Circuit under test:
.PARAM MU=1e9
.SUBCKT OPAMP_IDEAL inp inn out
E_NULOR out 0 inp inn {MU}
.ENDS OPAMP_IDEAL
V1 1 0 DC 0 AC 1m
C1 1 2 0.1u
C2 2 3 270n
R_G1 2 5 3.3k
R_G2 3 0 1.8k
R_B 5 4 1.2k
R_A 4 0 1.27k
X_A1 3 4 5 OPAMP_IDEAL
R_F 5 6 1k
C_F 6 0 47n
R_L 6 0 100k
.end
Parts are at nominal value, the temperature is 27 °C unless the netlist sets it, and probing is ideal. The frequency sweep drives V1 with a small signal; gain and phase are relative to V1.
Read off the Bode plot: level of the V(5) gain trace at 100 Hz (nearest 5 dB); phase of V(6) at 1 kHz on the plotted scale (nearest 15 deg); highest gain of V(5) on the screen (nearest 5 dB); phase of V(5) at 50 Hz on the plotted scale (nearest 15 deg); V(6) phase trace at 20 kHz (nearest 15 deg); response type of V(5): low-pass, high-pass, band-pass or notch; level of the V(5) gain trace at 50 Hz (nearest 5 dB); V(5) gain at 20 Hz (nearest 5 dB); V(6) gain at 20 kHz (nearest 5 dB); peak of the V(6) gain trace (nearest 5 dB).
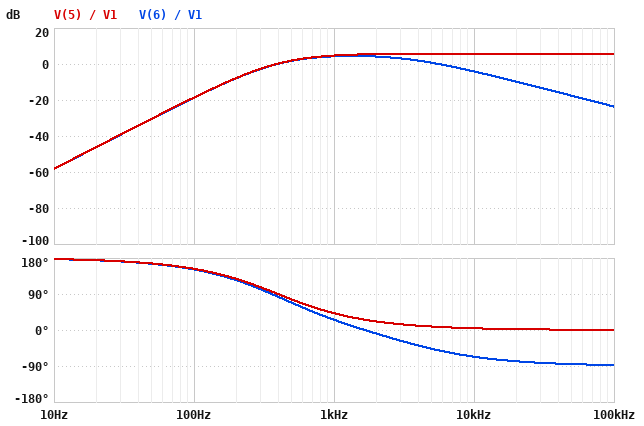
-20 dB
30 deg
5 dB
165 deg
-75 deg
high-pass
-30 dB
-45 dB
-10 dB
5 dB
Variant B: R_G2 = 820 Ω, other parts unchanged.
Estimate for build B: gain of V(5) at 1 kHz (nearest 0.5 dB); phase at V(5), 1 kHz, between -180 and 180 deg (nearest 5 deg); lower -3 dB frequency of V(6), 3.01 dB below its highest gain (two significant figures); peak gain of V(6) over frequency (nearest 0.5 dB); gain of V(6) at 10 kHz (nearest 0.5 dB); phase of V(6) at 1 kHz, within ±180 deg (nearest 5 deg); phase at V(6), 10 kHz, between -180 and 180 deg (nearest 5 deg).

-1.5 dB
75 deg
1.1 kHz
1.5 dB
-4.5 dB
55 deg
-60 deg
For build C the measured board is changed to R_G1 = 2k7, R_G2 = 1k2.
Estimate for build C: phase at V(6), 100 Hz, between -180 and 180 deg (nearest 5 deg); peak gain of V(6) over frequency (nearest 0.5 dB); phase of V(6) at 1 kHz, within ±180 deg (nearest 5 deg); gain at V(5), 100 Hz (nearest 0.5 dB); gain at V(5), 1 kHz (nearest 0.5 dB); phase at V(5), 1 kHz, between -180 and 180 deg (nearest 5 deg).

155 deg
3.5 dB
45 deg
-24.0 dB
2.5 dB
60 deg
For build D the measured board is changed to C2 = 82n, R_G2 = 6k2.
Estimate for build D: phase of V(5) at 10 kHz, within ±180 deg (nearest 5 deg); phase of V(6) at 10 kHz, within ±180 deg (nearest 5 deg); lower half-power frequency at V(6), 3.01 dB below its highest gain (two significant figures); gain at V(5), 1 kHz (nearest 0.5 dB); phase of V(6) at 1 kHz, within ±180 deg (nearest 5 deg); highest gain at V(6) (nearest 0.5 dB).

0 deg
-70 deg
350 Hz
7.0 dB
-10 deg
16.5 dB
